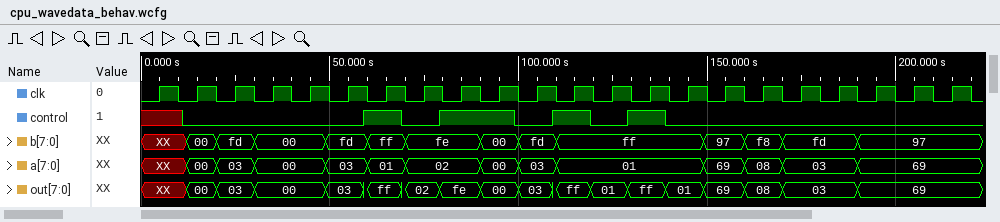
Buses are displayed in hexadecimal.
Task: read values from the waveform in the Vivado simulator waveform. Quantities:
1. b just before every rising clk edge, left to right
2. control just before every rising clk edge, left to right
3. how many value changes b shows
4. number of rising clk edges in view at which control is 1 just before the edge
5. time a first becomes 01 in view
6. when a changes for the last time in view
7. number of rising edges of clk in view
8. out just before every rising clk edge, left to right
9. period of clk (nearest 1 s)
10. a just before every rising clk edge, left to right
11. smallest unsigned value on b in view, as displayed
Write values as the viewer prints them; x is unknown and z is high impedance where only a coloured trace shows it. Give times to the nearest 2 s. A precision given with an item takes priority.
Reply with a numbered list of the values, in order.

1. XX, 00, fd, 00, 00, fd, ff, fe, fe, 00, fd, ff, ff, ff, ff, 97, f8, fd, fd, 97, 97, 97
2. x 0 0 0 0 0 1 0 1 1 0 1 0 1 0 0 0 0 0 0 0 0
3. 13
4. 5
5. 60 s
6. 190 s
7. 22
8. XX, 00, 03, 00, 00, 03, ff, 02, fe, 00, 03, ff, 01, ff, 01, 69, 08, 03, 03, 69, 69, 69
9. 10 s
10. XX, 00, 03, 00, 00, 03, 01, 02, 02, 00, 03, 01, 01, 01, 01, 69, 08, 03, 03, 69, 69, 69
11. 00
